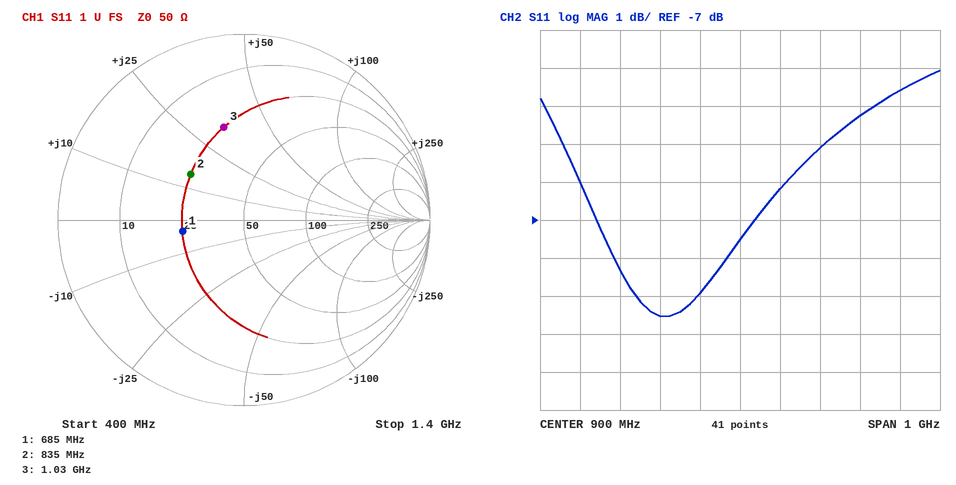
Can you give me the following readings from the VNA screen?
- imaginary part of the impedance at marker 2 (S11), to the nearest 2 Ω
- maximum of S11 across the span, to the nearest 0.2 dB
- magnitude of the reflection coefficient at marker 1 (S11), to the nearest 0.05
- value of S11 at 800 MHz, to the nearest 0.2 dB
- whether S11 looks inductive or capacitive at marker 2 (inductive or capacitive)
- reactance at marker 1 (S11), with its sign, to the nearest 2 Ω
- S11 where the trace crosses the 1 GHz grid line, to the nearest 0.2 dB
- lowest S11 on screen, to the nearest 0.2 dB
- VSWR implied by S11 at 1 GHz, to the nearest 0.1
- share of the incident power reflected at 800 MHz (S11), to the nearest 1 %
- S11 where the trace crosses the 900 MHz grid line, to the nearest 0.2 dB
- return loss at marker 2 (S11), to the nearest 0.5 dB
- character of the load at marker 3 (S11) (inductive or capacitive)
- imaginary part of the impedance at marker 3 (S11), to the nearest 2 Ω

+14 Ω
-3.0 dB
0.35
-9.0 dB
inductive
-4 Ω
-6.2 dB
-9.6 dB
2.9
13 %
-7.6 dB
8.5 dB
inductive
+34 Ω
